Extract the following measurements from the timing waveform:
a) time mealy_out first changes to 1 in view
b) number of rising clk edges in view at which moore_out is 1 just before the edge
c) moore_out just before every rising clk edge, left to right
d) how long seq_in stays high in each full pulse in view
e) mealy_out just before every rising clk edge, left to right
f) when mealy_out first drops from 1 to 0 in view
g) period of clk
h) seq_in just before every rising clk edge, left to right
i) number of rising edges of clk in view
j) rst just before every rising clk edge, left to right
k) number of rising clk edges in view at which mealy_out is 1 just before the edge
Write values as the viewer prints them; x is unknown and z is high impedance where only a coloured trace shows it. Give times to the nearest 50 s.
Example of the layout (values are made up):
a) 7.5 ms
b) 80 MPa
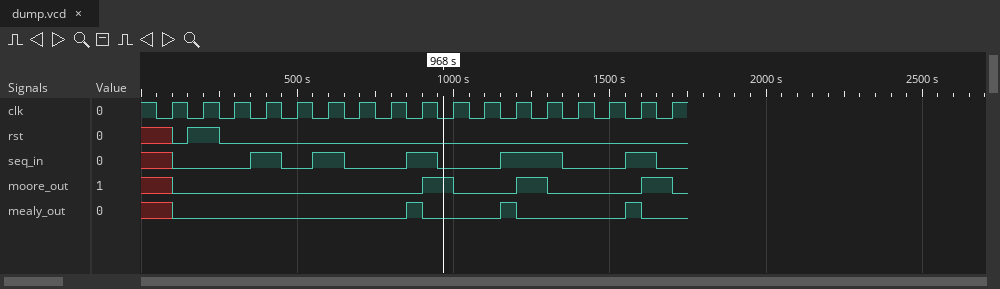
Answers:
a) 850 s
b) 3
c) x 0 0 0 0 0 0 0 0 1 0 0 1 0 0 0 1
d) 100 s, 100 s, 100 s, 200 s, 100 s
e) x 0 0 0 0 0 0 0 1 0 0 1 0 0 0 1 0
f) 900 s
g) 100 s
h) x 0 0 1 0 1 0 0 1 0 0 1 1 0 0 1 0
i) 17
j) x 1 0 0 0 0 0 0 0 0 0 0 0 0 0 0 0
k) 3
